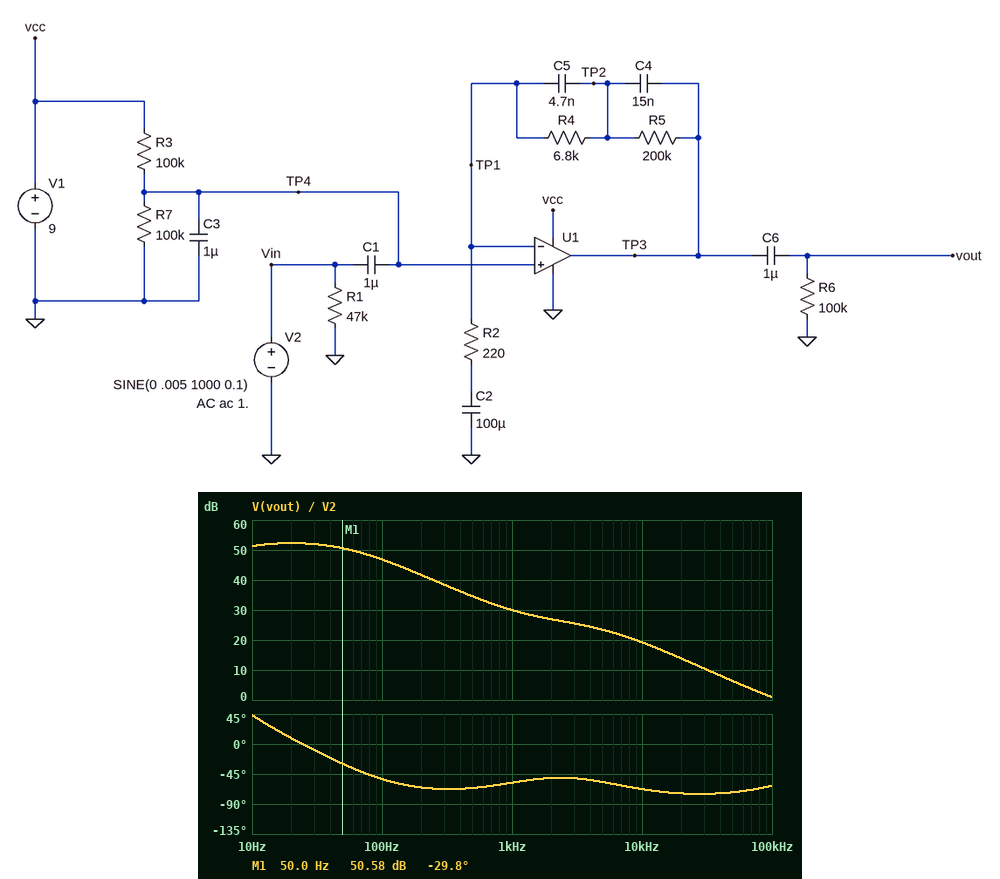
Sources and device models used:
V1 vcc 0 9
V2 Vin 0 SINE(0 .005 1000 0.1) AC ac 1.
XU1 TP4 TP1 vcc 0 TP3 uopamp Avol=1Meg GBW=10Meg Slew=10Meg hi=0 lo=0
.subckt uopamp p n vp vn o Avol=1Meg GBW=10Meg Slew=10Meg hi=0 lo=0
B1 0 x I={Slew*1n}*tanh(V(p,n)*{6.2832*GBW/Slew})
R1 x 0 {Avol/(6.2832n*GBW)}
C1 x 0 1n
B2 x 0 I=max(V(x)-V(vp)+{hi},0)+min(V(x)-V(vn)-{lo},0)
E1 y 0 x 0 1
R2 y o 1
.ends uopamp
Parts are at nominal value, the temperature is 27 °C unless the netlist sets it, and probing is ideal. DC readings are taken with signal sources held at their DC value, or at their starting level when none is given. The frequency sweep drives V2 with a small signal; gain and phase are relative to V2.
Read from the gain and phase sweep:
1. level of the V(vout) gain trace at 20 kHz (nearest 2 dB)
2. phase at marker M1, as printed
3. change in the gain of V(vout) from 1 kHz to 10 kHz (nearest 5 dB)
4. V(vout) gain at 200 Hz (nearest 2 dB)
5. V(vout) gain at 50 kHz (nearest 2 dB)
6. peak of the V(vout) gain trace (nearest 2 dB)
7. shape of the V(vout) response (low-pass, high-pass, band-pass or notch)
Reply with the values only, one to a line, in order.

14 dB
-29.8 deg
-10 dB
42 dB
6 dB
52 dB
low-pass
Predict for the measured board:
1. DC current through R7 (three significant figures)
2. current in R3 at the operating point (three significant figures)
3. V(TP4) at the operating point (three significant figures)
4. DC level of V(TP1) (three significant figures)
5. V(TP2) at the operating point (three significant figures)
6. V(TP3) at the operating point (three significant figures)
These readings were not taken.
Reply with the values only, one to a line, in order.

45.0 µA
45.0 µA
4.50 V
4.50 V
4.50 V
4.50 V
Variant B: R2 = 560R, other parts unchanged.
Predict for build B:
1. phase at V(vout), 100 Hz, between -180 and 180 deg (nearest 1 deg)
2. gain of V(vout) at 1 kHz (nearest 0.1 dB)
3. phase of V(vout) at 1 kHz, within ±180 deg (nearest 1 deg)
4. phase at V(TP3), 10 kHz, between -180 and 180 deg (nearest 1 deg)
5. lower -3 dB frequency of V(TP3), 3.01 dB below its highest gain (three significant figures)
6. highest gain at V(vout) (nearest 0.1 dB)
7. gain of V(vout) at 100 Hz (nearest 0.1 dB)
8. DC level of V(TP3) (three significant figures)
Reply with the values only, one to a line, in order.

-55 deg
22.0 dB
-57 deg
-63 deg
3.18 Hz
44.8 dB
38.8 dB
4.50 V
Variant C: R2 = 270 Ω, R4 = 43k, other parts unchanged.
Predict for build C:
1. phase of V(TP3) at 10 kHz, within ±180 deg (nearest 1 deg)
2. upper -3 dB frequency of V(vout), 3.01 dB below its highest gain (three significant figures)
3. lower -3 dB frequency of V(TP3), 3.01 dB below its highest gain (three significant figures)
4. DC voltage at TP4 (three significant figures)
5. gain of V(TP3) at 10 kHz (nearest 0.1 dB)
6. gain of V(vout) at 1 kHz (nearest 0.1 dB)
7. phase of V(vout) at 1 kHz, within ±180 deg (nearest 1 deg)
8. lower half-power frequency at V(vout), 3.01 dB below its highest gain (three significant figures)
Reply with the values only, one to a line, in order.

-83 deg
68.4 Hz
5.27 Hz
4.50 V
18.2 dB
36.4 dB
-61 deg
5.59 Hz
